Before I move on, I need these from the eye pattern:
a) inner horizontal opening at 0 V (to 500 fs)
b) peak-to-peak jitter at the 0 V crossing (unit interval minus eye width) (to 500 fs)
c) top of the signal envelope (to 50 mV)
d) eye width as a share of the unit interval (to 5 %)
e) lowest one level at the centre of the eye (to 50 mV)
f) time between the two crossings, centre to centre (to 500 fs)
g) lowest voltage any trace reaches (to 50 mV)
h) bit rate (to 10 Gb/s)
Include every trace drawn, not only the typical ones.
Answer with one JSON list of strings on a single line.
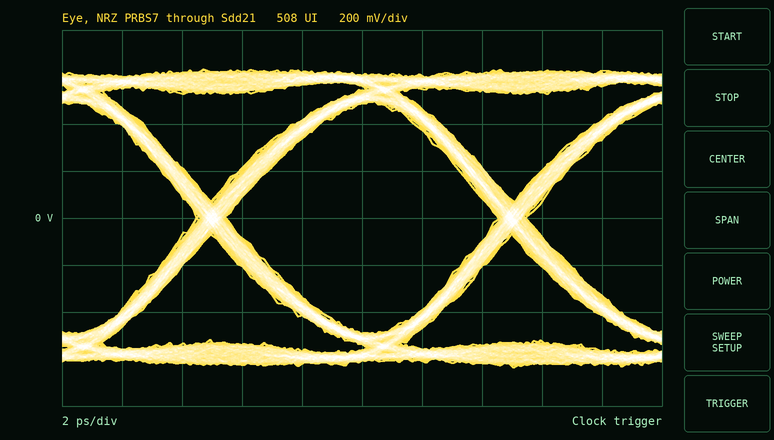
["9.0 ps", "1.0 ps", "650 mV", "90 %", "500 mV", "10.0 ps", "-650 mV", "100 Gb/s"]
